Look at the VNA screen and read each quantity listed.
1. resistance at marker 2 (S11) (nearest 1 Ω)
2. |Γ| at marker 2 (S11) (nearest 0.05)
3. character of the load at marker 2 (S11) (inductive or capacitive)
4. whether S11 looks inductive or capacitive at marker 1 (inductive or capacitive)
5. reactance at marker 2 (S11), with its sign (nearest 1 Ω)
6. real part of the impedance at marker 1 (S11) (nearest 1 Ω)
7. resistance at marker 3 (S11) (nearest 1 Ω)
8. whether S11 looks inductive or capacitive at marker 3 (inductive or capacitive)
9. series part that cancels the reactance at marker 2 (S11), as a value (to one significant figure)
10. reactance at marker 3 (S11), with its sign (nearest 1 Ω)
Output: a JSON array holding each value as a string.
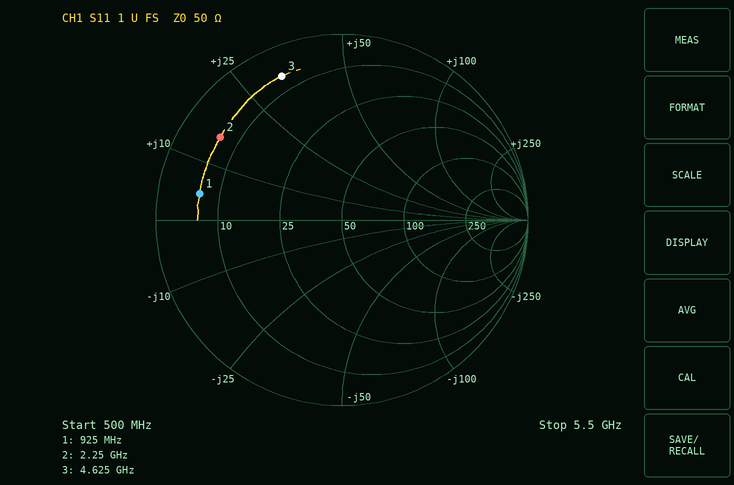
["6 Ω", "0.80", "inductive", "inductive", "+15 Ω", "6 Ω", "6 Ω", "inductive", "5 pF", "+33 Ω"]
